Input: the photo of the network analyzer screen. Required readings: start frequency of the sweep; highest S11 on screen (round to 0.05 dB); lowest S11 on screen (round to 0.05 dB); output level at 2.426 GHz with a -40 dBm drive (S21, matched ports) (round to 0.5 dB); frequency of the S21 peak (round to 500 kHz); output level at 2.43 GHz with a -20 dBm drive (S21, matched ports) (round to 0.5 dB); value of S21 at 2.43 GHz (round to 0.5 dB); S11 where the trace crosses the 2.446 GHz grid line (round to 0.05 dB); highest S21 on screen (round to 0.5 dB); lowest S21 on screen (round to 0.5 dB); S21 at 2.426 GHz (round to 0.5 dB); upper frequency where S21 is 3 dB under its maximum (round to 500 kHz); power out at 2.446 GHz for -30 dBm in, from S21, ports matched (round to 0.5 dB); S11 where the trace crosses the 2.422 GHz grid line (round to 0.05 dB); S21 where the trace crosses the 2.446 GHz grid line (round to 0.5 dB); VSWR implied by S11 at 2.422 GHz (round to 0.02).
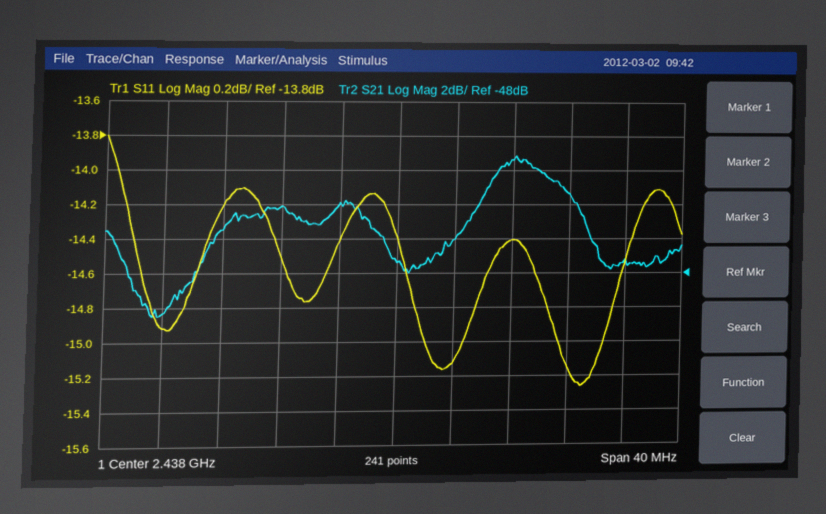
2.418 GHz
-13.80 dB
-15.25 dB
-85.5 dBm
2.4460 GHz
-64.0 dBm
-44.0 dB
-14.40 dB
-41.0 dB
-50.5 dB
-45.5 dB
2.4505 GHz
-71.5 dBm
-14.90 dB
-41.5 dB
1.44
